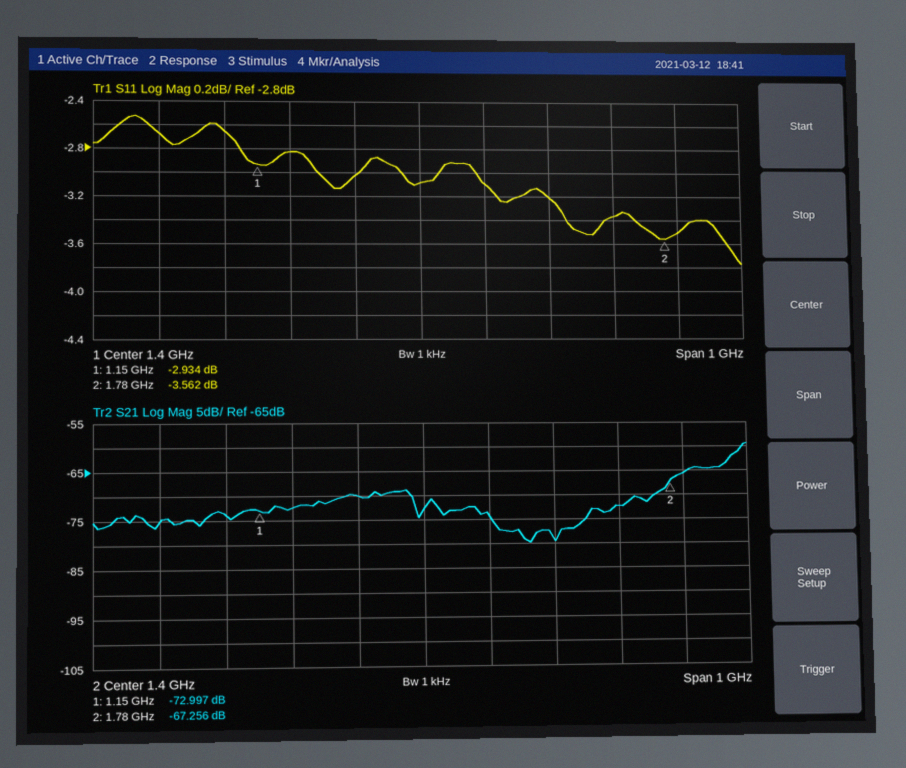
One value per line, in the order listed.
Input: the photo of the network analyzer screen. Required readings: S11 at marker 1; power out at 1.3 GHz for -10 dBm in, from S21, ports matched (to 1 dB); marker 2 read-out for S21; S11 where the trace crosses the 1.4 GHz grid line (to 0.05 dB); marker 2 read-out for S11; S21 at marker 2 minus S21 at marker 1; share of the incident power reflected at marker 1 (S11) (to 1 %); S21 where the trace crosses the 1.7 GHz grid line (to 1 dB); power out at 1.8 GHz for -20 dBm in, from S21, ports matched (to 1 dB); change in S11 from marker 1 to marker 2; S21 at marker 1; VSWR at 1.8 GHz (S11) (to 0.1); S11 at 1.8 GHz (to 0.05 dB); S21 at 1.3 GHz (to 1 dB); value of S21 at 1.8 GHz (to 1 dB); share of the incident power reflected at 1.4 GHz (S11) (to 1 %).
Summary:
-2.934 dB
-80 dBm
-67.256 dB
-3.10 dB
-3.562 dB
5.741 dB
51 %
-72 dB
-86 dBm
-0.628 dB
-72.997 dB
5.0
-3.50 dB
-70 dB
-66 dB
49 %
